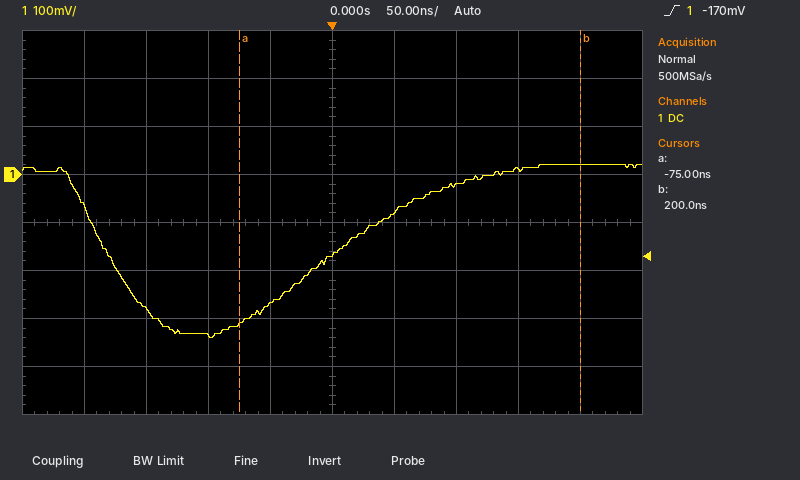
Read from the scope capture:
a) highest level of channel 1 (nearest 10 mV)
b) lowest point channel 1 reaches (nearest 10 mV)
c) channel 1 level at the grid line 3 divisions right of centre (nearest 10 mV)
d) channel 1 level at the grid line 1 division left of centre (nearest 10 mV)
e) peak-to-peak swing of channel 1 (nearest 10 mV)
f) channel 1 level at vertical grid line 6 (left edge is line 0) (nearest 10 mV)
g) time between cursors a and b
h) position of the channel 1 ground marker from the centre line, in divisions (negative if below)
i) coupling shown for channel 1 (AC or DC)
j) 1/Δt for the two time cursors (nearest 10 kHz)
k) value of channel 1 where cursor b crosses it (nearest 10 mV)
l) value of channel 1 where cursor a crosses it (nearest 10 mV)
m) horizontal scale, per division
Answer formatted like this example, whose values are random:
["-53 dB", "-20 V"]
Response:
["20 mV", "-340 mV", "10 mV", "-270 mV", "360 mV", "-80 mV", "275 ns", "+1.0 div", "DC", "3.64 MHz", "20 mV", "-310 mV", "50 ns"]
